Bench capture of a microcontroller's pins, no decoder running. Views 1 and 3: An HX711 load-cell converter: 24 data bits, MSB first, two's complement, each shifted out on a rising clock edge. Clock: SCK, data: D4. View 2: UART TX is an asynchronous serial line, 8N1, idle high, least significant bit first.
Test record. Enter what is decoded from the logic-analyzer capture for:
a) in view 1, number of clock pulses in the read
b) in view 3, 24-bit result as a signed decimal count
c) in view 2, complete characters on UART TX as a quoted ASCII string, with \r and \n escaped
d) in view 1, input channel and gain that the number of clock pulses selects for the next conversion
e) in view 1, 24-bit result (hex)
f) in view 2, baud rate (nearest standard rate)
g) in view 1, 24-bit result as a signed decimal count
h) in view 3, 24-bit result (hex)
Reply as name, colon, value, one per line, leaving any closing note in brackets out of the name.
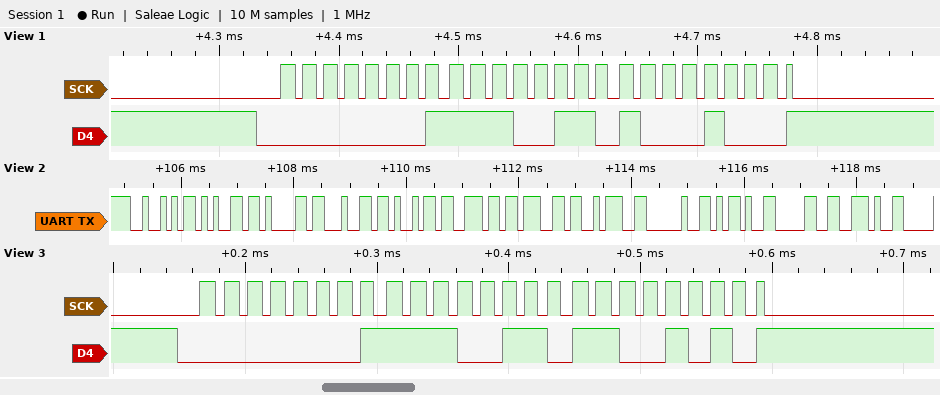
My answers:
in view 1, number of clock pulses in the read: 25
in view 3, 24-bit result as a signed decimal count: 124618
in view 2, complete characters on UART TX as a quoted ASCII string, with \r and \n escaped: "Reading: -0."
in view 1, input channel and gain that the number of clock pulses selects for the next conversion: channel A, gain 128
in view 1, 24-bit result: 0x01E688
in view 2, baud rate: 9600 baud
in view 1, 24-bit result as a signed decimal count: 124552
in view 3, 24-bit result: 0x01E6CA
